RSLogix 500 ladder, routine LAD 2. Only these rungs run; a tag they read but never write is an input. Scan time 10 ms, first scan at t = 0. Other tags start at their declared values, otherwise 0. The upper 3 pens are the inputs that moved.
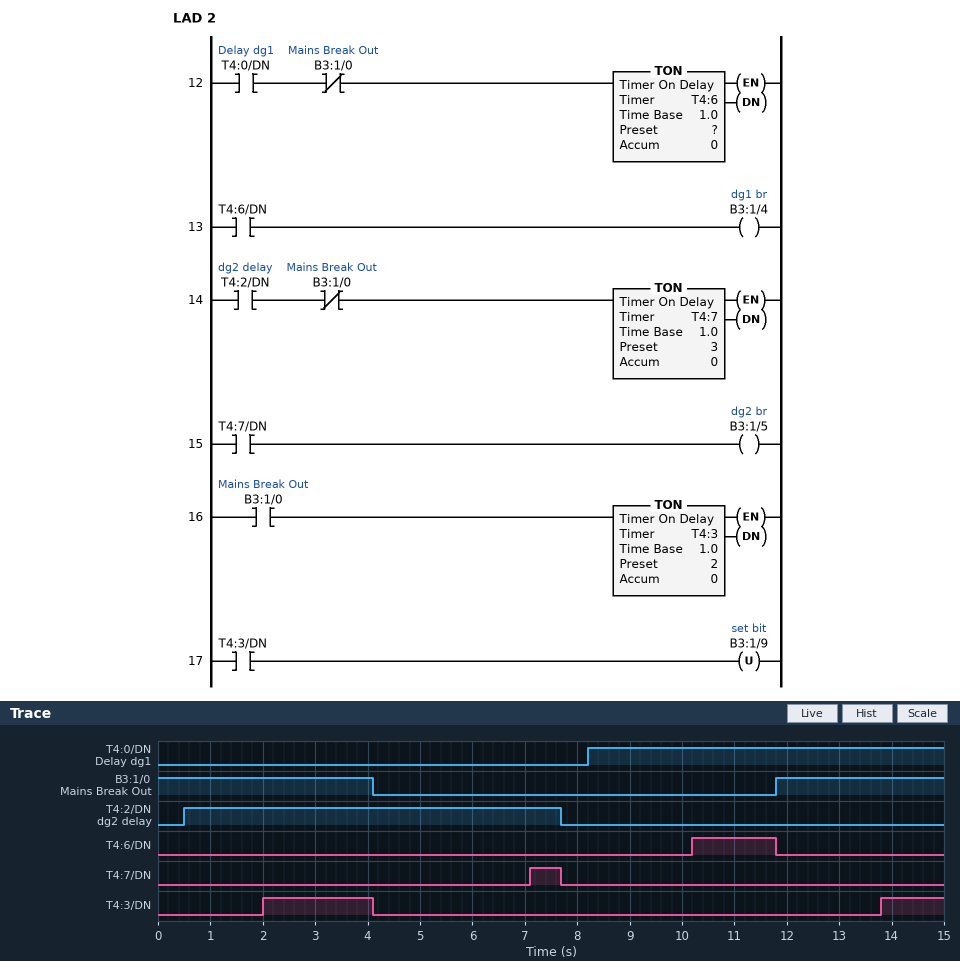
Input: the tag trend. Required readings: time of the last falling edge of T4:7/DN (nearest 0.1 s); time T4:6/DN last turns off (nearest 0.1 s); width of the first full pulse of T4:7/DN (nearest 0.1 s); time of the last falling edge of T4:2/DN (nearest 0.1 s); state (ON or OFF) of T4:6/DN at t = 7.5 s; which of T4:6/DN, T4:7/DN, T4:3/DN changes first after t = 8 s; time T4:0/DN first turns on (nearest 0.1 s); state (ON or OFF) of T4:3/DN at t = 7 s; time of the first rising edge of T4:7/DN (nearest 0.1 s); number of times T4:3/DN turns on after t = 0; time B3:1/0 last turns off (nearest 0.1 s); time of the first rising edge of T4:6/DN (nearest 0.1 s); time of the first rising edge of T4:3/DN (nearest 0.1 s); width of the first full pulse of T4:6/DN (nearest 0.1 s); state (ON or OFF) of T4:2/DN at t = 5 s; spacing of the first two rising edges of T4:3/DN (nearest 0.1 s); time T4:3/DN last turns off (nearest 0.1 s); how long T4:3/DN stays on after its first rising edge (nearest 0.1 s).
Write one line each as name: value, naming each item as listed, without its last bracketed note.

time of the last falling edge of T4:7/DN: 7.7 s
time T4:6/DN last turns off: 11.8 s
width of the first full pulse of T4:7/DN: 0.6 s
time of the last falling edge of T4:2/DN: 7.7 s
state (ON or OFF) of T4:6/DN at t = 7.5 s: OFF
which of T4:6/DN, T4:7/DN, T4:3/DN changes first after t = 8 s: T4:6/DN
time T4:0/DN first turns on: 8.2 s
state (ON or OFF) of T4:3/DN at t = 7 s: OFF
time of the first rising edge of T4:7/DN: 7.1 s
number of times T4:3/DN turns on after t = 0: 2
time B3:1/0 last turns off: 4.1 s
time of the first rising edge of T4:6/DN: 10.2 s
time of the first rising edge of T4:3/DN: 2.0 s
width of the first full pulse of T4:6/DN: 1.6 s
state (ON or OFF) of T4:2/DN at t = 5 s: ON
spacing of the first two rising edges of T4:3/DN: 11.8 s
time T4:3/DN last turns off: 4.1 s
how long T4:3/DN stays on after its first rising edge: 2.1 s
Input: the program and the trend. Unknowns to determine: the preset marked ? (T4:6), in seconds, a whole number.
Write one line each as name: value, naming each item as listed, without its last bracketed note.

the preset marked ? (T4:6), in seconds, a whole number: 2 s
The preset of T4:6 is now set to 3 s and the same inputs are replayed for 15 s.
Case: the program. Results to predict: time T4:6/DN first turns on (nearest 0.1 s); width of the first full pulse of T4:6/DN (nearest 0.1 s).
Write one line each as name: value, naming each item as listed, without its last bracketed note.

time T4:6/DN first turns on: 11.2 s
width of the first full pulse of T4:6/DN: 0.6 s
